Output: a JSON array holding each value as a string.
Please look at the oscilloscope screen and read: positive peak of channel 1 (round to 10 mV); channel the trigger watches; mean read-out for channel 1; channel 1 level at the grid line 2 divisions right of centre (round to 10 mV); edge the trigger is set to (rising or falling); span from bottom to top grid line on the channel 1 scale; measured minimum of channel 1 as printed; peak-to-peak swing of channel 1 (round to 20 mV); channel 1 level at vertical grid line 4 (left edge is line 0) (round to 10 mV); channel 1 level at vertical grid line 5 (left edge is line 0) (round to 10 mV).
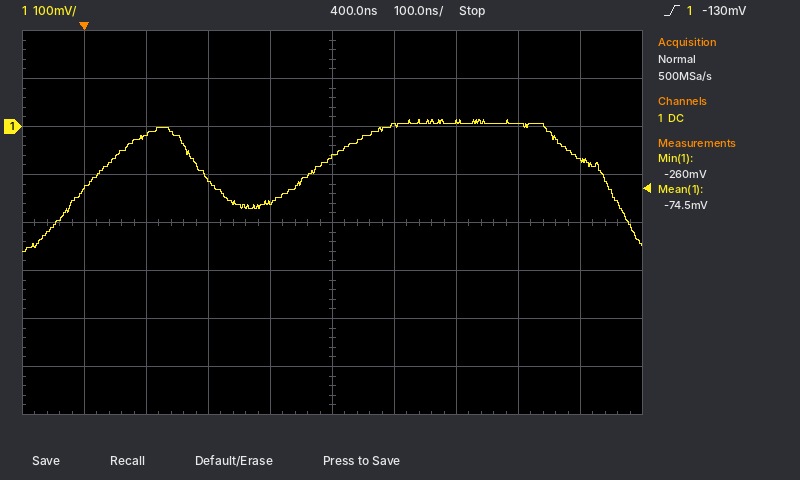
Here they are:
["10 mV", "channel 1", "-74.5 mV", "10 mV", "rising", "800 mV", "-260 mV", "280 mV", "-160 mV", "-60 mV"]
